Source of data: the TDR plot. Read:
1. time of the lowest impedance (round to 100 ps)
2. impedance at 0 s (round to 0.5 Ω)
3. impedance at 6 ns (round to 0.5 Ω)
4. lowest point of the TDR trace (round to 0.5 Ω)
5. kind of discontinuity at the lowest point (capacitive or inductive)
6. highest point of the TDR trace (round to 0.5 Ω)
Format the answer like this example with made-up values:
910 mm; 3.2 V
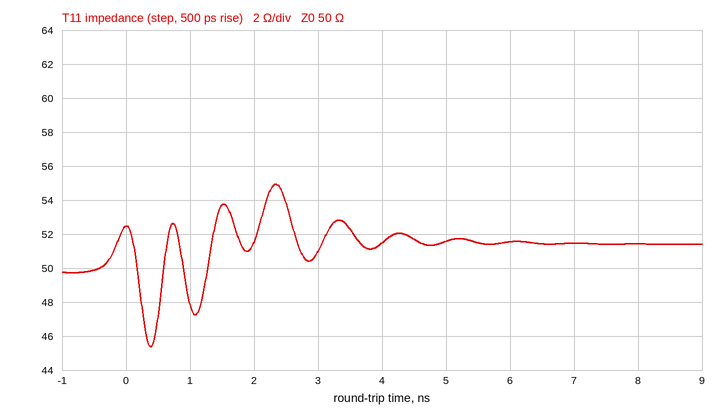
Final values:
400 ps; 52.5 Ω; 51.5 Ω; 45.5 Ω; capacitive; 55.0 Ω
